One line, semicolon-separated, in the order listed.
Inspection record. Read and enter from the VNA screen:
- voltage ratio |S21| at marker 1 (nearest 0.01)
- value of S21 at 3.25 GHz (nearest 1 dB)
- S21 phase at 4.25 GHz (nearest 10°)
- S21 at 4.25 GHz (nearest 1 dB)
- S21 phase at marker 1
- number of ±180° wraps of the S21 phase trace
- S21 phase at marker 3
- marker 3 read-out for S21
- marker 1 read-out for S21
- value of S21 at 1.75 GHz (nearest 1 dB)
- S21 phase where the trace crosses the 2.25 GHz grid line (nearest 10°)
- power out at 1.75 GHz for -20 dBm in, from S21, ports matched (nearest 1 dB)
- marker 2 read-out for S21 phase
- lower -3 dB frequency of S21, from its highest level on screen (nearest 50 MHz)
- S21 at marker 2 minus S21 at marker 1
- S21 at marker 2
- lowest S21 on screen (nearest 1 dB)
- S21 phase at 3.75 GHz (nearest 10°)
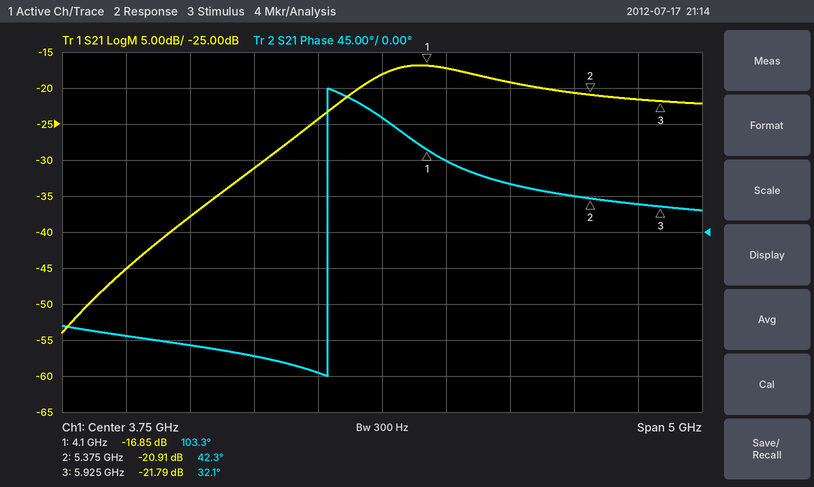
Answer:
0.14; -24 dB; 90°; -17 dB; 103.3°; 1; 32.1°; -21.79 dB; -16.85 dB; -45 dB; -140°; -65 dBm; 42.3°; 3.60 GHz; -4.06 dB; -20.91 dB; -54 dB; 140°
